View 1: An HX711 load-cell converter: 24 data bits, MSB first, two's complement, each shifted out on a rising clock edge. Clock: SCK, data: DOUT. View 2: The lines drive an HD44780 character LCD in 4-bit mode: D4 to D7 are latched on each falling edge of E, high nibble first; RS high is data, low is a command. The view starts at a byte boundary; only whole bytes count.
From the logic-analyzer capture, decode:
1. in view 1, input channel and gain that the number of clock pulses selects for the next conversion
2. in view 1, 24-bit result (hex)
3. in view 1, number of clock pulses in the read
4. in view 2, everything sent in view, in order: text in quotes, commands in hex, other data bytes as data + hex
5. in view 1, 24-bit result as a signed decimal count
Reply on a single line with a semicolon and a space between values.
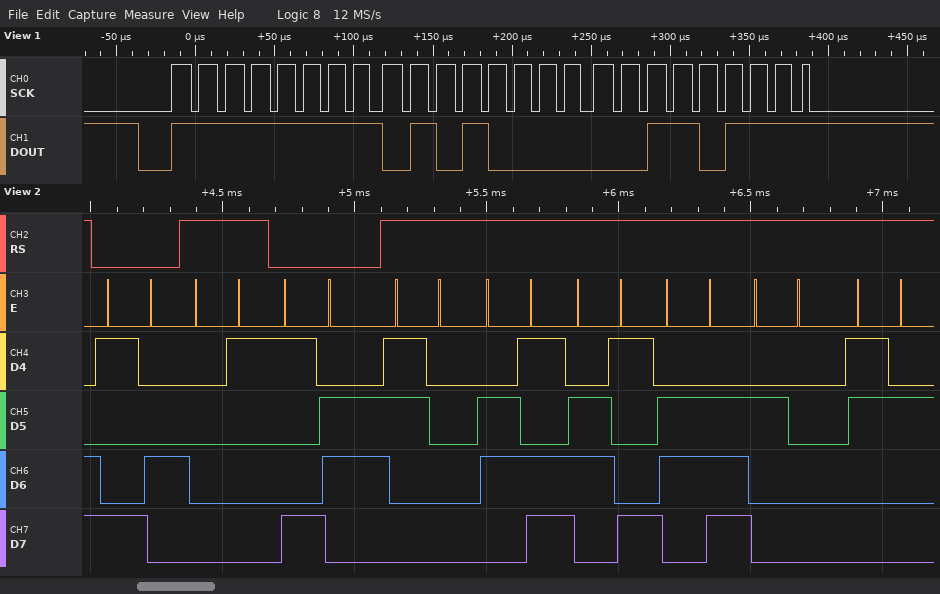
channel A, gain 128; 0xFF5037; 25; 0x94 data 01 0x96 "0min 2"; -45001
